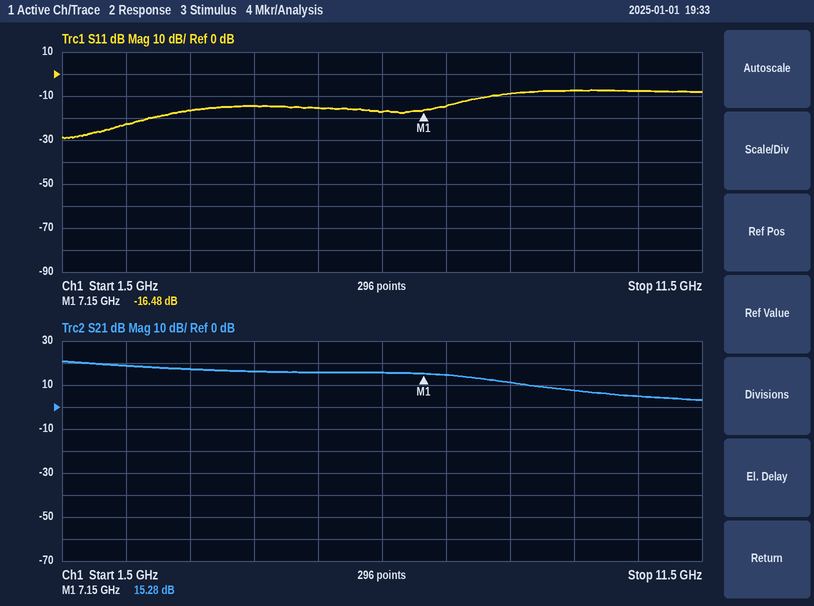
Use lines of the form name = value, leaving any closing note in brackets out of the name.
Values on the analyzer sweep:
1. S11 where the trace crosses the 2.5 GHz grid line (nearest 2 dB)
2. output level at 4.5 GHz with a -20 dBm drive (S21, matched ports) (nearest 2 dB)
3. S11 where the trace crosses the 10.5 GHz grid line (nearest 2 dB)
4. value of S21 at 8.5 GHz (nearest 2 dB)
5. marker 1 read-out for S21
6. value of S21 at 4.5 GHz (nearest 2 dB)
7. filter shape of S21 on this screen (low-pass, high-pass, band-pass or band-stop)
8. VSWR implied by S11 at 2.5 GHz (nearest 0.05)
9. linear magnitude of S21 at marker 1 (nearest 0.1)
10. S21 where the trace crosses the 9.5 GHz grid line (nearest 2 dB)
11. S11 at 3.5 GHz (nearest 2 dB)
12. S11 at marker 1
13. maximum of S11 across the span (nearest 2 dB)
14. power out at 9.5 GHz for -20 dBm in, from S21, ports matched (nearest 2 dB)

S11 where the trace crosses the 2.5 GHz grid line = -22 dB
output level at 4.5 GHz with a -20 dBm drive (S21, matched ports) = -4 dBm
S11 where the trace crosses the 10.5 GHz grid line = -8 dB
value of S21 at 8.5 GHz = 12 dB
marker 1 read-out for S21 = 15.28 dB
value of S21 at 4.5 GHz = 16 dB
filter shape of S21 on this screen = low-pass
VSWR implied by S11 at 2.5 GHz = 1.15
linear magnitude of S21 at marker 1 = 5.8
S21 where the trace crosses the 9.5 GHz grid line = 8 dB
S11 at 3.5 GHz = -16 dB
S11 at marker 1 = -16.48 dB
maximum of S11 across the span = -8 dB
power out at 9.5 GHz for -20 dBm in, from S21, ports matched = -12 dBm
